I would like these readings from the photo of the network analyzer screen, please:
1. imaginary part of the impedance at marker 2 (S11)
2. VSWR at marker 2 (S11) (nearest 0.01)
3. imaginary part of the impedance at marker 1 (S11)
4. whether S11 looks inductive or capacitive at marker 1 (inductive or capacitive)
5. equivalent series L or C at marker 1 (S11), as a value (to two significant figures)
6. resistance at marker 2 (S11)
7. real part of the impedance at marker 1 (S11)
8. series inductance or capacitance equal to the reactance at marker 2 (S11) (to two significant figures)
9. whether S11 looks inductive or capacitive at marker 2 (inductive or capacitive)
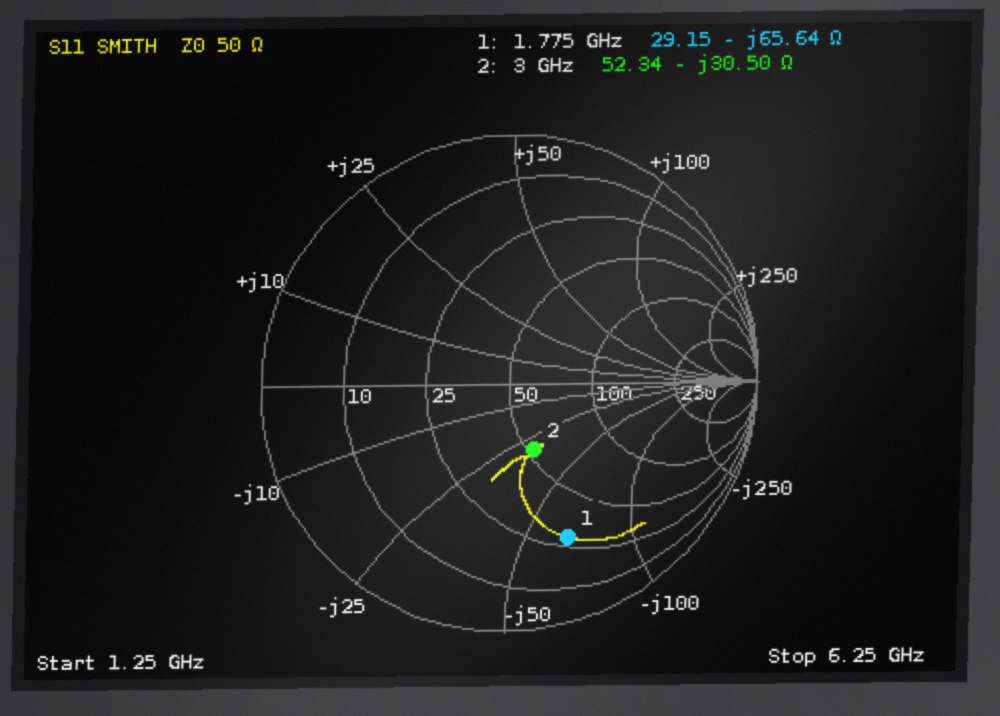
-30.50 Ω
1.80
-65.64 Ω
capacitive
1.4 pF
52.34 Ω
29.15 Ω
1.7 pF
capacitive
